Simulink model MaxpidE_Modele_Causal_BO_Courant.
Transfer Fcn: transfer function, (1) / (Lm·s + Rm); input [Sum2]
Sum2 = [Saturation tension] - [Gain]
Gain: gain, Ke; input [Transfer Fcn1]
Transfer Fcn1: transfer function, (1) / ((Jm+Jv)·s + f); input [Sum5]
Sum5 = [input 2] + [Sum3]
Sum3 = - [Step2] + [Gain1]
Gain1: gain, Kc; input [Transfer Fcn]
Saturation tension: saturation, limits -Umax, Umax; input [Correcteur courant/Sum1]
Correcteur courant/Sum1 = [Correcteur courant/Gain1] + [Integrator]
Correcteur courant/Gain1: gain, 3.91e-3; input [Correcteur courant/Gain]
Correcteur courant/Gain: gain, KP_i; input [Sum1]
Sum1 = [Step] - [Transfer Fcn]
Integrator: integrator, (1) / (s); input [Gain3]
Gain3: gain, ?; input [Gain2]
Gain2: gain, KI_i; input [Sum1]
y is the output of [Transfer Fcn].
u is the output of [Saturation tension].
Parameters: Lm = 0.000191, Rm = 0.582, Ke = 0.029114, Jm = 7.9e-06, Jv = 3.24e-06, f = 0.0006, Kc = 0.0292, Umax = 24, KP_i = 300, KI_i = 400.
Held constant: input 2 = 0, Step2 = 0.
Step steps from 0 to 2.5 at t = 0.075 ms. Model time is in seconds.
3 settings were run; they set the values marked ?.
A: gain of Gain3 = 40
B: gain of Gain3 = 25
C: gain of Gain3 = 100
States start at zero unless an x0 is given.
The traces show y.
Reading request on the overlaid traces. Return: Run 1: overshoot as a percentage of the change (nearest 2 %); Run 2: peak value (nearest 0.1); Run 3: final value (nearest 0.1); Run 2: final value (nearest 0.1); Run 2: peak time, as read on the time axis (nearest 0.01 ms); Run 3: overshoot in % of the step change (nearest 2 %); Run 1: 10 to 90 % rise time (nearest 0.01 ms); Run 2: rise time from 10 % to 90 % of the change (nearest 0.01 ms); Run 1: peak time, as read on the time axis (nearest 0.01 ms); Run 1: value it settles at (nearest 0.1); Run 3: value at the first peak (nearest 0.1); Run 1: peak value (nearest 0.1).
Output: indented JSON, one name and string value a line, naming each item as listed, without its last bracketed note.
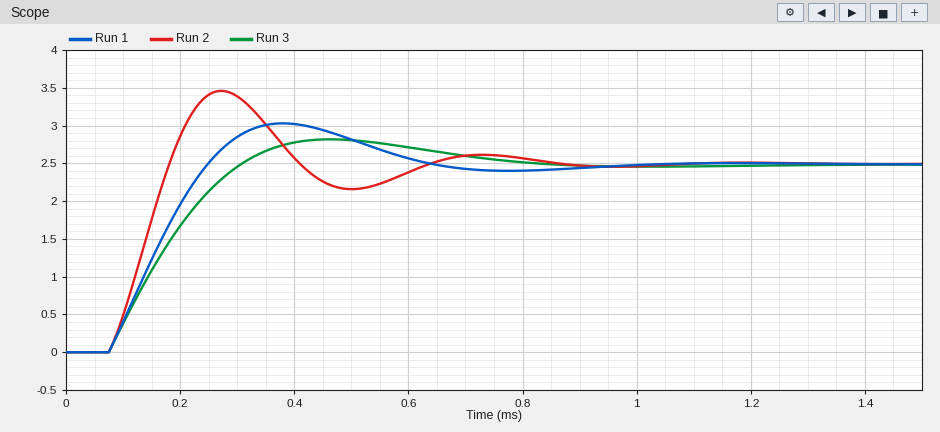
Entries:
{
  "Run 1: overshoot as a percentage of the change": "22 %",
  "Run 2: peak value": "3.5",
  "Run 3: final value": "2.5",
  "Run 2: final value": "2.5",
  "Run 2: peak time, as read on the time axis": "0.27 ms",
  "Run 3: overshoot in % of the step change": "14 %",
  "Run 1: 10 to 90 % rise time": "0.13 ms",
  "Run 2: rise time from 10 % to 90 % of the change": "0.08 ms",
  "Run 1: peak time, as read on the time axis": "0.38 ms",
  "Run 1: value it settles at": "2.5",
  "Run 3: value at the first peak": "2.8",
  "Run 1: peak value": "3.0"
}
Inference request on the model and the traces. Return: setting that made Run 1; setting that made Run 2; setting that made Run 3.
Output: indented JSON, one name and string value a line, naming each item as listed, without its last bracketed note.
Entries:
{
  "setting that made Run 1": "A",
  "setting that made Run 2": "C",
  "setting that made Run 3": "B"
}
